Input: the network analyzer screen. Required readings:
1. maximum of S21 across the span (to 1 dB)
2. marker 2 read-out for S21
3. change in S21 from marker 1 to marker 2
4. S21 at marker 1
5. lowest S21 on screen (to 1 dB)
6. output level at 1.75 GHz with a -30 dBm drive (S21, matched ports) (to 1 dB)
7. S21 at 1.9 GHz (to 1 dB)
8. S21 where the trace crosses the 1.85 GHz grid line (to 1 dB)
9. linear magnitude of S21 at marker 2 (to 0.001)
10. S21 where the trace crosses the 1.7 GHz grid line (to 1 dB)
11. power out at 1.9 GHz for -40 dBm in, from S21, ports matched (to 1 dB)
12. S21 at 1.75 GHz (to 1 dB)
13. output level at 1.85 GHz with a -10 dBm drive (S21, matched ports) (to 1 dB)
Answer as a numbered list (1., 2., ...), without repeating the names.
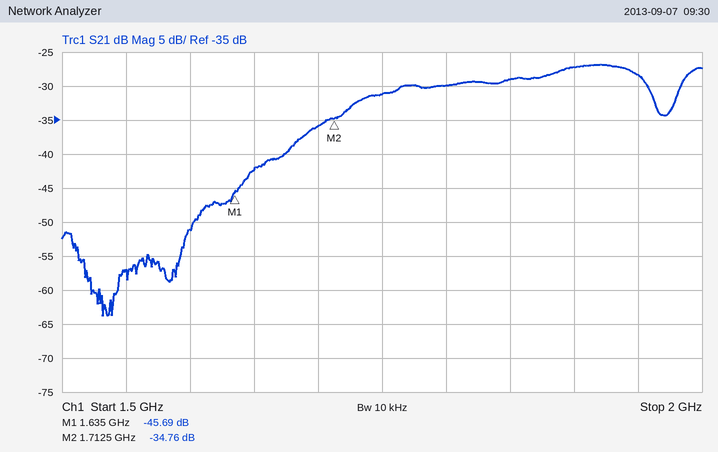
1. -27 dB
2. -34.76 dB
3. 10.93 dB
4. -45.69 dB
5. -64 dB
6. -61 dBm
7. -27 dB
8. -29 dB
9. 0.018
10. -36 dB
11. -67 dBm
12. -31 dB
13. -39 dBm
